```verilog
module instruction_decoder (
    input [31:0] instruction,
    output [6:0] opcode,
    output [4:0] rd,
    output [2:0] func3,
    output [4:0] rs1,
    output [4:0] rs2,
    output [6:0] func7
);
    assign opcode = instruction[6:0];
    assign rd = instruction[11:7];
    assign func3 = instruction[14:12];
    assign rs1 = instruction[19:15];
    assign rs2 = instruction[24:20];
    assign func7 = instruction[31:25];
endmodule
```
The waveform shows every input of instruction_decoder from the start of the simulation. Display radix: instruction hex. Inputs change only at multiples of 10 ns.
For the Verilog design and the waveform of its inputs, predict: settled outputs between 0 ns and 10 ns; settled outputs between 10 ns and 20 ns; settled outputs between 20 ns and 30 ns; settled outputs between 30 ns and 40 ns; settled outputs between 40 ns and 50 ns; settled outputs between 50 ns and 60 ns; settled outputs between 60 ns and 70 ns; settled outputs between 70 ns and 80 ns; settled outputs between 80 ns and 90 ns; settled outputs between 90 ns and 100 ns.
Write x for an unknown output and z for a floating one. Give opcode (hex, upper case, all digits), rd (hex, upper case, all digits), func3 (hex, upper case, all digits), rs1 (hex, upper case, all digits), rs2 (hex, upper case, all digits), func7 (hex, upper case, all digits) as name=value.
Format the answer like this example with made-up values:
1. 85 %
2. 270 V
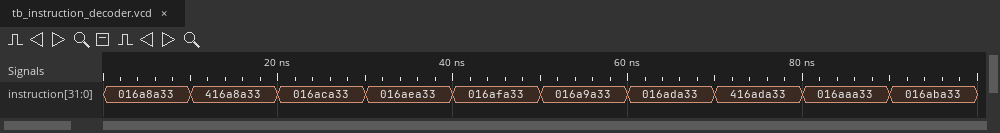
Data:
1. opcode=33, rd=14, func3=0, rs1=15, rs2=16, func7=00
2. opcode=33, rd=14, func3=0, rs1=15, rs2=16, func7=20
3. opcode=33, rd=14, func3=4, rs1=15, rs2=16, func7=00
4. opcode=33, rd=14, func3=6, rs1=15, rs2=16, func7=00
5. opcode=33, rd=14, func3=7, rs1=15, rs2=16, func7=00
6. opcode=33, rd=14, func3=1, rs1=15, rs2=16, func7=00
7. opcode=33, rd=14, func3=5, rs1=15, rs2=16, func7=00
8. opcode=33, rd=14, func3=5, rs1=15, rs2=16, func7=20
9. opcode=33, rd=14, func3=2, rs1=15, rs2=16, func7=00
10. opcode=33, rd=14, func3=3, rs1=15, rs2=16, func7=00
